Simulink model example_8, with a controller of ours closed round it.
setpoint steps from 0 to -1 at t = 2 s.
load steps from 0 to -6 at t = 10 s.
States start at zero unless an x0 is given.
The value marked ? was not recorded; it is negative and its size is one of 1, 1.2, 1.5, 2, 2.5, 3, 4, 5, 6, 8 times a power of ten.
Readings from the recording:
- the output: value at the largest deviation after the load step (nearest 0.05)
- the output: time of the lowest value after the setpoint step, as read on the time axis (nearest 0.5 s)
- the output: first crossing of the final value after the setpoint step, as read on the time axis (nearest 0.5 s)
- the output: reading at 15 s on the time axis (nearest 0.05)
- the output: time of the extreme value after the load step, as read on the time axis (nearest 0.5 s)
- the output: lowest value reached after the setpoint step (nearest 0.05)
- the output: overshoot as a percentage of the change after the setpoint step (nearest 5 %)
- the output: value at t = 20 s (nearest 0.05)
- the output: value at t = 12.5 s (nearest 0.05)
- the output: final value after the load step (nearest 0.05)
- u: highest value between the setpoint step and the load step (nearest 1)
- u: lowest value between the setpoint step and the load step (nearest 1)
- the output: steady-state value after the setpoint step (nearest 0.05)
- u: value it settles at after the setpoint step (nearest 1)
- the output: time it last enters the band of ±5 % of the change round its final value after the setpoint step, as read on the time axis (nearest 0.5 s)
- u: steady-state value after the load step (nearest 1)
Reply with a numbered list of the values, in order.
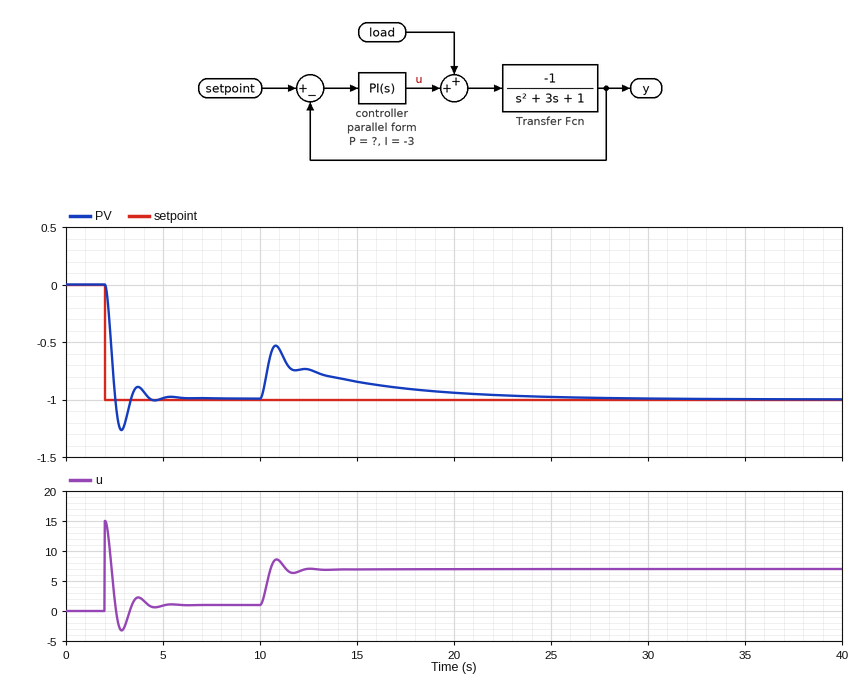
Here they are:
1. -0.55
2. 3.0 s
3. 2.5 s
4. -0.85
5. 11.0 s
6. -1.25
7. 25 %
8. -0.95
9. -0.75
10. -1.00
11. 15
12. -3
13. -1.00
14. 1
15. 4.0 s
16. 7
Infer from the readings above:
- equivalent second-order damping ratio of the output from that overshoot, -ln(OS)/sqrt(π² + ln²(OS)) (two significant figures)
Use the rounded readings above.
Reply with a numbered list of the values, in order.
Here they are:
1. 0.40
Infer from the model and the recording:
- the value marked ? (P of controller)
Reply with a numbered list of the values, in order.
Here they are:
1. -15
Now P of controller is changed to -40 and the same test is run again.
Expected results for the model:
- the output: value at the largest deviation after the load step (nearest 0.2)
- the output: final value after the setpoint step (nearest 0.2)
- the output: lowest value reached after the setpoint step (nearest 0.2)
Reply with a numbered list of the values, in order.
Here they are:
1. -0.8
2. -1.0
3. -1.4
